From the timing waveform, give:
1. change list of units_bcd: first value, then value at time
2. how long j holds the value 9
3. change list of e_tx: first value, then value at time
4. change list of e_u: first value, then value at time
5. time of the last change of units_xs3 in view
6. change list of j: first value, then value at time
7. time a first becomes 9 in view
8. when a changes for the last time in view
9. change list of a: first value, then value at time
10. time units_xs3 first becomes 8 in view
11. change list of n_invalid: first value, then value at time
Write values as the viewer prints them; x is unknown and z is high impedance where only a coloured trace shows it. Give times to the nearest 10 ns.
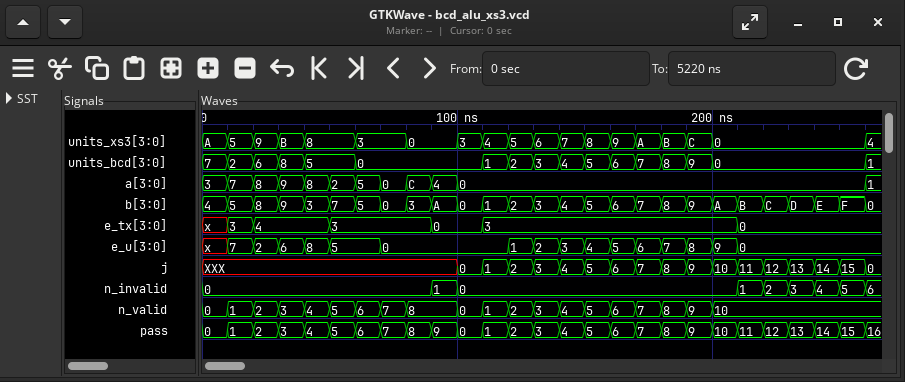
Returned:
7, 2 at 10 ns, 6 at 20 ns, 8 at 30 ns, 5 at 40 ns, 0 at 60 ns, 1 at 110 ns, 2 at 120 ns, 3 at 130 ns, 4 at 140 ns, 5 at 150 ns, 6 at 160 ns, 7 at 170 ns, 8 at 180 ns, 9 at 190 ns, 0 at 200 ns, 1 at 260 ns
10 ns
x, 3 at 10 ns, 4 at 20 ns, 3 at 50 ns, 0 at 90 ns, 3 at 110 ns, 0 at 210 ns
x, 7 at 10 ns, 2 at 20 ns, 6 at 30 ns, 8 at 40 ns, 5 at 50 ns, 0 at 70 ns, 1 at 120 ns, 2 at 130 ns, 3 at 140 ns, 4 at 150 ns, 5 at 160 ns, 6 at 170 ns, 7 at 180 ns, 8 at 190 ns, 9 at 200 ns, 0 at 210 ns
260 ns
XXX, 0 at 100 ns, 1 at 110 ns, 2 at 120 ns, 3 at 130 ns, 4 at 140 ns, 5 at 150 ns, 6 at 160 ns, 7 at 170 ns, 8 at 180 ns, 9 at 190 ns, 10 at 200 ns, 11 at 210 ns, 12 at 220 ns, 13 at 230 ns, 14 at 240 ns, 15 at 250 ns, 0 at 260 ns
30 ns
260 ns
3, 7 at 10 ns, 8 at 20 ns, 9 at 30 ns, 8 at 40 ns, 2 at 50 ns, 5 at 60 ns, 0 at 70 ns, C at 80 ns, 4 at 90 ns, 0 at 100 ns, 1 at 260 ns
40 ns
0, 1 at 90 ns, 0 at 100 ns, 1 at 210 ns, 2 at 220 ns, 3 at 230 ns, 4 at 240 ns, 5 at 250 ns, 6 at 260 ns
